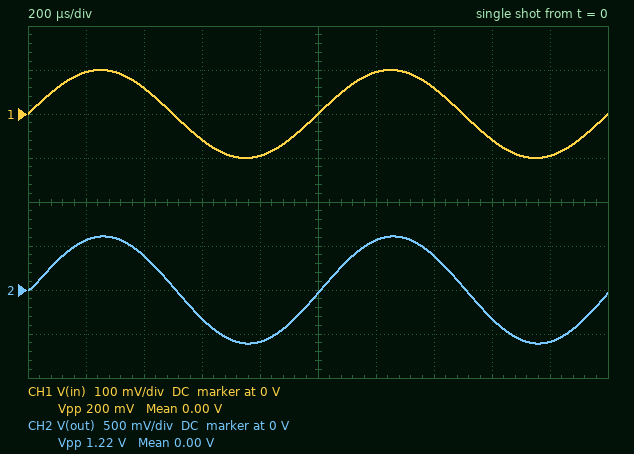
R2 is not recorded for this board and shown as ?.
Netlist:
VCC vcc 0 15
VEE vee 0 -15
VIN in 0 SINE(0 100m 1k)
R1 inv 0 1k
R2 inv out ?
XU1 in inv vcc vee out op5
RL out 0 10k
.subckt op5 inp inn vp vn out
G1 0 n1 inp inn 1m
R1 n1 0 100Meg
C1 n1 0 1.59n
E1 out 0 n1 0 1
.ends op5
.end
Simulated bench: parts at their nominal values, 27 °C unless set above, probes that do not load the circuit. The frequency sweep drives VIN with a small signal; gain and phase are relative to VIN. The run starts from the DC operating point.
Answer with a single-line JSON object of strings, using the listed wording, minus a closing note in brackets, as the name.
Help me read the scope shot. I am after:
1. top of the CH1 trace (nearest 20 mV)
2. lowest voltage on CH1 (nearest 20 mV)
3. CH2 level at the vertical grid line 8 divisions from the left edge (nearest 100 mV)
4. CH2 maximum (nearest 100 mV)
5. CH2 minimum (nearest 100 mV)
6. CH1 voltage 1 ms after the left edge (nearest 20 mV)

{"top of the CH1 trace": "100 mV", "lowest voltage on CH1": "-100 mV", "CH2 level at the vertical grid line 8 divisions from the left edge": "-300 mV", "CH2 maximum": "600 mV", "CH2 minimum": "-600 mV", "CH1 voltage 1 ms after the left edge": "0 V"}
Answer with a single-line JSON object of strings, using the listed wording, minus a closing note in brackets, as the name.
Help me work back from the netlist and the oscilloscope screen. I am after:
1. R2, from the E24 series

{"R2, from the E24 series": "5.1 kΩ"}
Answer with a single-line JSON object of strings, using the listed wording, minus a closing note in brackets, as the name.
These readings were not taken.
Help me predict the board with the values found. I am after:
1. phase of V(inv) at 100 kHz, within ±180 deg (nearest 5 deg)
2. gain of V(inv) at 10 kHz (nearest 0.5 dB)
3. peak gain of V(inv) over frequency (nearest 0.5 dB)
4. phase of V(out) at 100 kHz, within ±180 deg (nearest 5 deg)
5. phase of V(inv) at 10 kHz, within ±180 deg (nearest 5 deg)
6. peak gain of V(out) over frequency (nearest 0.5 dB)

{"phase of V(inv) at 100 kHz, within ±180 deg": "-80 deg", "gain of V(inv) at 10 kHz": "-1.5 dB", "peak gain of V(inv) over frequency": "0 dB", "phase of V(out) at 100 kHz, within ±180 deg": "-80 deg", "phase of V(inv) at 10 kHz, within ±180 deg": "-30 deg", "peak gain of V(out) over frequency": "15.5 dB"}
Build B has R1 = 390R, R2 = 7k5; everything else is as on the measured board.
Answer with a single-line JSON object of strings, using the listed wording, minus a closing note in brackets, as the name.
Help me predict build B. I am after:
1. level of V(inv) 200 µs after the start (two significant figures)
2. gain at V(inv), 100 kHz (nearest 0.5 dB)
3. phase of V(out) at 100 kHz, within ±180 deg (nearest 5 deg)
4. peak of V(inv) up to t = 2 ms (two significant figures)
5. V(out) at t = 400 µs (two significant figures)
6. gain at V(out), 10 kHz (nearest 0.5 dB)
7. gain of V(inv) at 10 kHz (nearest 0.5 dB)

{"level of V(inv) 200 µs after the start": "85 mV", "gain at V(inv), 100 kHz": "-26.0 dB", "phase of V(out) at 100 kHz, within ±180 deg": "-85 deg", "peak of V(inv) up to t = 2 ms": "98 mV", "V(out) at t = 400 µs": "1.5 V", "gain at V(out), 10 kHz": "19.0 dB", "gain of V(inv) at 10 kHz": "-7.0 dB"}
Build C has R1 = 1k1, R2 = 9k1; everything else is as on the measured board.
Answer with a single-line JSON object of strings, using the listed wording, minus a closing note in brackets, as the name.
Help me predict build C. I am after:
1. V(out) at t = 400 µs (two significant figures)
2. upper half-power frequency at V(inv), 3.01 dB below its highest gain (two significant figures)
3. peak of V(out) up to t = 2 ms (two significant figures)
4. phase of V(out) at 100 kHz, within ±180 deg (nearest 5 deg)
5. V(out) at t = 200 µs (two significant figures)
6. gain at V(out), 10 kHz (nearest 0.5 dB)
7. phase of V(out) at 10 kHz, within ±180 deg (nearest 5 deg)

{"V(out) at t = 400 µs": "610 mV", "upper half-power frequency at V(inv), 3.01 dB below its highest gain": "11 kHz", "peak of V(out) up to t = 2 ms": "920 mV", "phase of V(out) at 100 kHz, within ±180 deg": "-85 deg", "V(out) at t = 200 µs": "850 mV", "gain at V(out), 10 kHz": "16.5 dB", "phase of V(out) at 10 kHz, within ±180 deg": "-45 deg"}
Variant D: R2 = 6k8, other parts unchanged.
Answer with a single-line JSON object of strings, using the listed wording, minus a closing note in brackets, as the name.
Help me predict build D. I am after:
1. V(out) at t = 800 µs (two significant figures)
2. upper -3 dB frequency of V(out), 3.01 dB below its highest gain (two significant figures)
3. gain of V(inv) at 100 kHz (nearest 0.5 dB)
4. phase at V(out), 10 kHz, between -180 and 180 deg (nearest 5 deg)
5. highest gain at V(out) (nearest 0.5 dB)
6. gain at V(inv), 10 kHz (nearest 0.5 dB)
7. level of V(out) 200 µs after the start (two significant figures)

{"V(out) at t = 800 µs": "-760 mV", "upper -3 dB frequency of V(out), 3.01 dB below its highest gain": "13 kHz", "gain of V(inv) at 100 kHz": "-18.0 dB", "phase at V(out), 10 kHz, between -180 and 180 deg": "-40 deg", "highest gain at V(out)": "18.0 dB", "gain at V(inv), 10 kHz": "-2.0 dB", "level of V(out) 200 µs after the start": "720 mV"}
